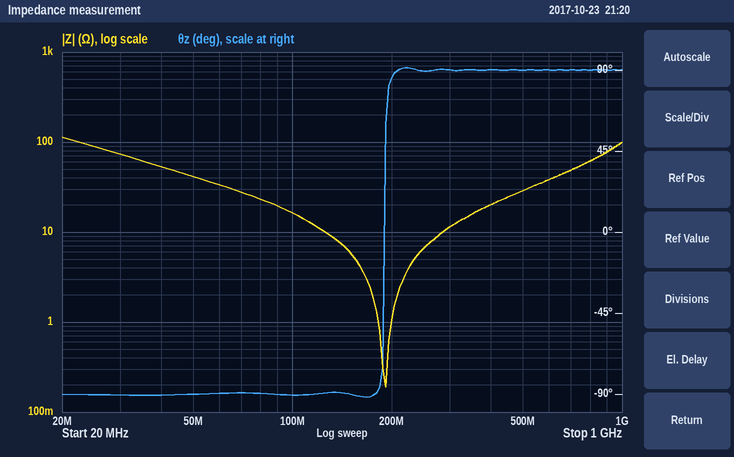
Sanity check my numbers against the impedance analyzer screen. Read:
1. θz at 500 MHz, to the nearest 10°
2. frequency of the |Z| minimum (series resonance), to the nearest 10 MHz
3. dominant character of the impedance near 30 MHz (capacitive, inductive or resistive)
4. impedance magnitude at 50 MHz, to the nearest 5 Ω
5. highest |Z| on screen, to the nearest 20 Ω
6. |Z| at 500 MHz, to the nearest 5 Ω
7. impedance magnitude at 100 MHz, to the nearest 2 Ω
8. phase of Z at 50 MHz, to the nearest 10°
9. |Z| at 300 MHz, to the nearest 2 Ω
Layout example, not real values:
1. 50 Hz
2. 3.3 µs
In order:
1. 90°
2. 190 MHz
3. capacitive
4. 40 Ω
5. 120 Ω
6. 30 Ω
7. 16 Ω
8. -90°
9. 12 Ω
